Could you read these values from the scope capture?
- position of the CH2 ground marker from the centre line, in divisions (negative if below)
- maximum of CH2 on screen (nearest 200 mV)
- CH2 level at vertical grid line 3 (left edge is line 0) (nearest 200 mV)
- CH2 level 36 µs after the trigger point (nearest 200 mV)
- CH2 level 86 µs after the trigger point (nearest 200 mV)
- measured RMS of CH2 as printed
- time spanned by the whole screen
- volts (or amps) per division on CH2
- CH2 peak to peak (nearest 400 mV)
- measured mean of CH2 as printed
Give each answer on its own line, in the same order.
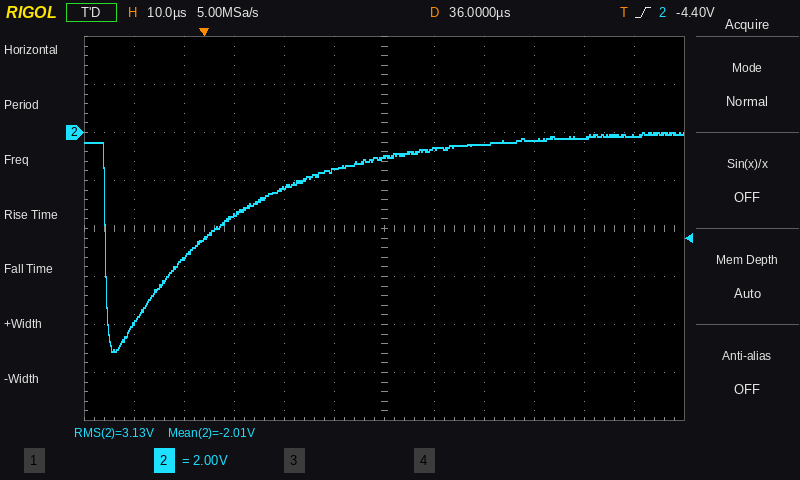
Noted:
+2.0 div
0.0 V
-3.4 V
-1.0 V
-200 mV
3.13 V
120 µs
2 V
9.2 V
-2.01 V
